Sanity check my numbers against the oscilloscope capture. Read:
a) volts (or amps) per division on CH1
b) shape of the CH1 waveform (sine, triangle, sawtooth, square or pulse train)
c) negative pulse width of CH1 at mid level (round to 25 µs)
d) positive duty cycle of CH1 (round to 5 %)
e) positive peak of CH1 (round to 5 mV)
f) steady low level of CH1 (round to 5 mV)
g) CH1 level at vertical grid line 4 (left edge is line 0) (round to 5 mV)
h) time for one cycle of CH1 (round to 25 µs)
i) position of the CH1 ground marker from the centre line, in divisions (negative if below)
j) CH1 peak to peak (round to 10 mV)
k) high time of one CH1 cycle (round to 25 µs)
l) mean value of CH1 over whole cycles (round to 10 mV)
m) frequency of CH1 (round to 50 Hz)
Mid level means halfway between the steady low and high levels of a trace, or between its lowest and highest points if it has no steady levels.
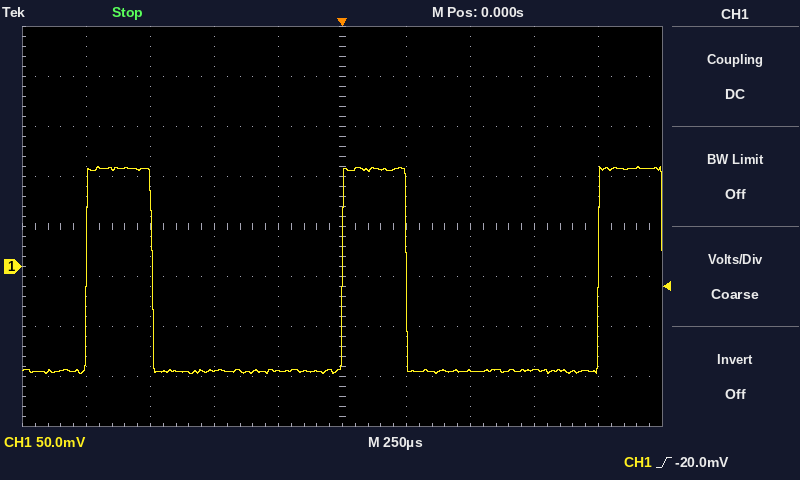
50 mV
pulse train
750 µs
25 %
100 mV
-105 mV
-105 mV
1.000 ms
-0.8 div
210 mV
250 µs
-50 mV
1.00 kHz
